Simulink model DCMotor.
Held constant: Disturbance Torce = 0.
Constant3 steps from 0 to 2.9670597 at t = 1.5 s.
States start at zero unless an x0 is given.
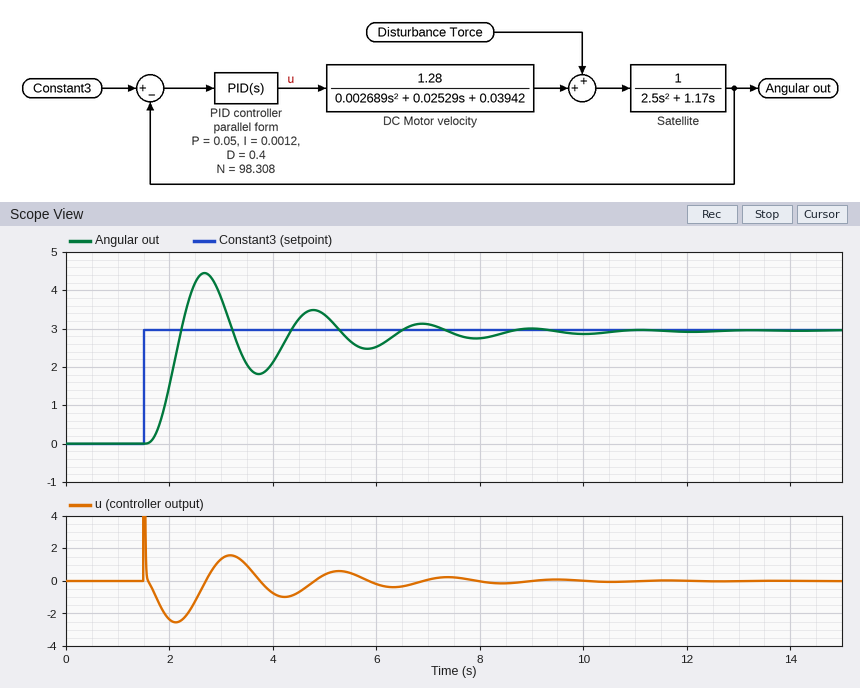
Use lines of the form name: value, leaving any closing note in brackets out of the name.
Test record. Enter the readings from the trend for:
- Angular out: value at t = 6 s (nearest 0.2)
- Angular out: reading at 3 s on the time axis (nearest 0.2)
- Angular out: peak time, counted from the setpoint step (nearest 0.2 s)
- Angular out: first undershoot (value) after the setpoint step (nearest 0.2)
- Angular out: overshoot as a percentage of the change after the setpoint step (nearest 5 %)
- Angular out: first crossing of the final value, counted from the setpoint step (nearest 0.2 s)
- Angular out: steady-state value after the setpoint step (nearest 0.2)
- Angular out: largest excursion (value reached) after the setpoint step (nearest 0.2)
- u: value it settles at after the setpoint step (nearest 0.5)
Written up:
Angular out: value at t = 6 s: 2.6
Angular out: reading at 3 s on the time axis: 3.8
Angular out: peak time, counted from the setpoint step: 1.2 s
Angular out: first undershoot (value) after the setpoint step: 1.8
Angular out: overshoot as a percentage of the change after the setpoint step: 50 %
Angular out: first crossing of the final value, counted from the setpoint step: 0.8 s
Angular out: steady-state value after the setpoint step: 3.0
Angular out: largest excursion (value reached) after the setpoint step: 4.4
u: value it settles at after the setpoint step: 0.0
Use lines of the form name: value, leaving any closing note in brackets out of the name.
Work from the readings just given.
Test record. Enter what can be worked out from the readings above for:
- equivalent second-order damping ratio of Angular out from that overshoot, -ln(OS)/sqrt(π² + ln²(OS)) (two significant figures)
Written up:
equivalent second-order damping ratio of Angular out from that overshoot, -ln(OS)/sqrt(π² + ln²(OS)): 0.22
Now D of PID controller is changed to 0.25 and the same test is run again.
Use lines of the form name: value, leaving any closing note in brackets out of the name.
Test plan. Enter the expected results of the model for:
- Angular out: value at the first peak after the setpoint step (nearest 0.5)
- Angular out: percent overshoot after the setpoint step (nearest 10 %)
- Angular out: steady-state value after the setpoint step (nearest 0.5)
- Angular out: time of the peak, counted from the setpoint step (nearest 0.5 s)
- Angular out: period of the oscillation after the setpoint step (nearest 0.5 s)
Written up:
Angular out: value at the first peak after the setpoint step: 4.0
Angular out: percent overshoot after the setpoint step: 30 %
Angular out: steady-state value after the setpoint step: 3.0
Angular out: time of the peak, counted from the setpoint step: 1.5 s
Angular out: period of the oscillation after the setpoint step: 2.5 s
